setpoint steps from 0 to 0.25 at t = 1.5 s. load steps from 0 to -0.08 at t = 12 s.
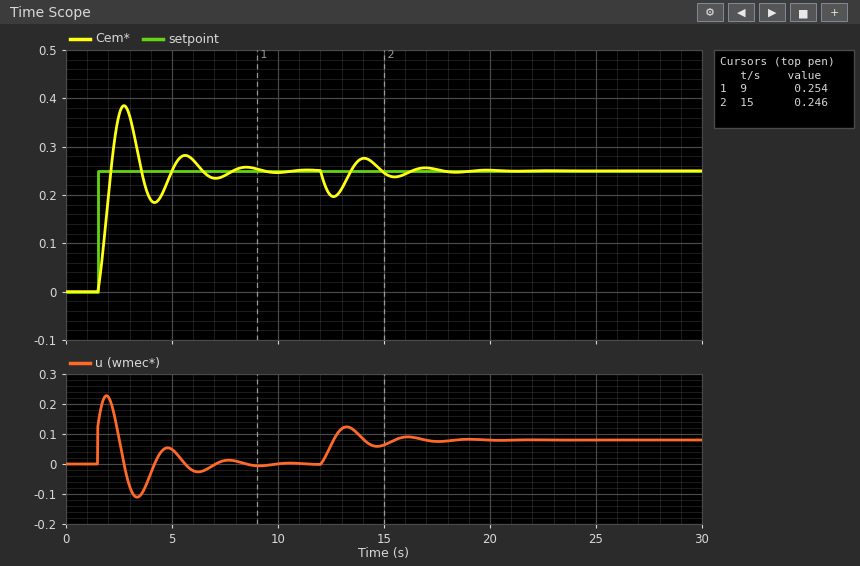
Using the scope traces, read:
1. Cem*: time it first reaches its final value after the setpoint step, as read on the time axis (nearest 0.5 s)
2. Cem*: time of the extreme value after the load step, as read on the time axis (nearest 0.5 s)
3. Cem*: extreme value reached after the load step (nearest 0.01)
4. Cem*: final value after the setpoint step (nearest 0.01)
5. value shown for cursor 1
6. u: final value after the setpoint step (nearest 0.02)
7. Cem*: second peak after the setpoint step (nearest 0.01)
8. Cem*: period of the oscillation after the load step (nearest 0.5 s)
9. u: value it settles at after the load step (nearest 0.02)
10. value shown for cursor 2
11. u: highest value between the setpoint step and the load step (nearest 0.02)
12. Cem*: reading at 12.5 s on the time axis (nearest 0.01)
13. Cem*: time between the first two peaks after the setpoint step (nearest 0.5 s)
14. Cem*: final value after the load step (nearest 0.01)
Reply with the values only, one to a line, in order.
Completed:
2.0 s
12.5 s
0.20
0.25
0.254
0.00
0.28
3.0 s
0.08
0.246
0.22
0.20
3.0 s
0.25
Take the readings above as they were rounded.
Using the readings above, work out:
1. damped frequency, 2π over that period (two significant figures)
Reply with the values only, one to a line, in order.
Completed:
2.1 rad/s
